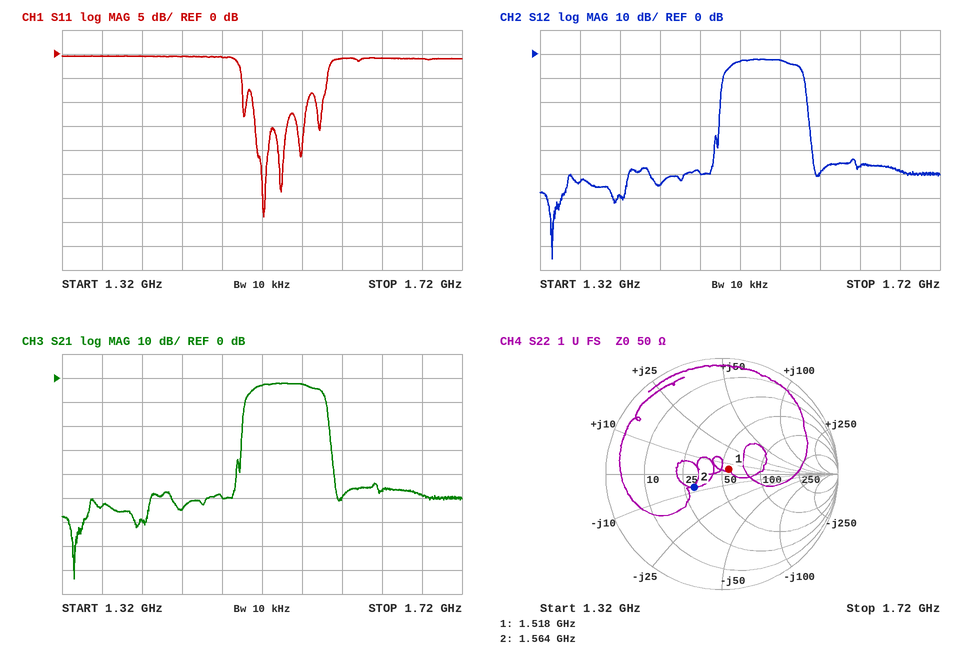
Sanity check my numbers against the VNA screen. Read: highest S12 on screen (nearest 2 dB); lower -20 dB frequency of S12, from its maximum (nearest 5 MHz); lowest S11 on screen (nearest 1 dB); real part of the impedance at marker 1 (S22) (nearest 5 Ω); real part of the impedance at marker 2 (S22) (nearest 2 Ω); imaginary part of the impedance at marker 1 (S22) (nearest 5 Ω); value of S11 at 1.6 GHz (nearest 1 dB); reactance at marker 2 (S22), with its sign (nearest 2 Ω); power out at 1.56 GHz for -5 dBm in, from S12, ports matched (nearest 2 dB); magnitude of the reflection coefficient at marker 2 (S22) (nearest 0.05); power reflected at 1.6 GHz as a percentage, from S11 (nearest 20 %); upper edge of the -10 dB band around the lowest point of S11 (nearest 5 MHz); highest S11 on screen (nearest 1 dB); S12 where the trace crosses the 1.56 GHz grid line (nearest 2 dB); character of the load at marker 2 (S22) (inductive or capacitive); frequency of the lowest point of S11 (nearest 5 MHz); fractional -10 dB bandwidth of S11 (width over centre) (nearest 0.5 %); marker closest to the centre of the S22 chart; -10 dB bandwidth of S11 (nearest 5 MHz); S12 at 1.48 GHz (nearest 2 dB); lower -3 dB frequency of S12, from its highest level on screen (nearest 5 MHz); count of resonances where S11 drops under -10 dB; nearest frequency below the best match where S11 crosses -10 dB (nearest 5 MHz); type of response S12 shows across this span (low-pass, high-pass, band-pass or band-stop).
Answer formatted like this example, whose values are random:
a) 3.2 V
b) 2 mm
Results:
a) -2 dB
b) 1.500 GHz
c) -34 dB
d) 55 Ω
e) 30 Ω
f) +5 Ω
g) -1 dB
h) -8 Ω
i) -8 dBm
j) 0.25
k) 80 %
l) 1.565 GHz
m) 0 dB
n) -2 dB
o) capacitive
p) 1.520 GHz
q) 3.5 %
r) marker 1
s) 55 MHz
t) -50 dB
u) 1.510 GHz
v) 5
w) 1.510 GHz
x) band-pass
